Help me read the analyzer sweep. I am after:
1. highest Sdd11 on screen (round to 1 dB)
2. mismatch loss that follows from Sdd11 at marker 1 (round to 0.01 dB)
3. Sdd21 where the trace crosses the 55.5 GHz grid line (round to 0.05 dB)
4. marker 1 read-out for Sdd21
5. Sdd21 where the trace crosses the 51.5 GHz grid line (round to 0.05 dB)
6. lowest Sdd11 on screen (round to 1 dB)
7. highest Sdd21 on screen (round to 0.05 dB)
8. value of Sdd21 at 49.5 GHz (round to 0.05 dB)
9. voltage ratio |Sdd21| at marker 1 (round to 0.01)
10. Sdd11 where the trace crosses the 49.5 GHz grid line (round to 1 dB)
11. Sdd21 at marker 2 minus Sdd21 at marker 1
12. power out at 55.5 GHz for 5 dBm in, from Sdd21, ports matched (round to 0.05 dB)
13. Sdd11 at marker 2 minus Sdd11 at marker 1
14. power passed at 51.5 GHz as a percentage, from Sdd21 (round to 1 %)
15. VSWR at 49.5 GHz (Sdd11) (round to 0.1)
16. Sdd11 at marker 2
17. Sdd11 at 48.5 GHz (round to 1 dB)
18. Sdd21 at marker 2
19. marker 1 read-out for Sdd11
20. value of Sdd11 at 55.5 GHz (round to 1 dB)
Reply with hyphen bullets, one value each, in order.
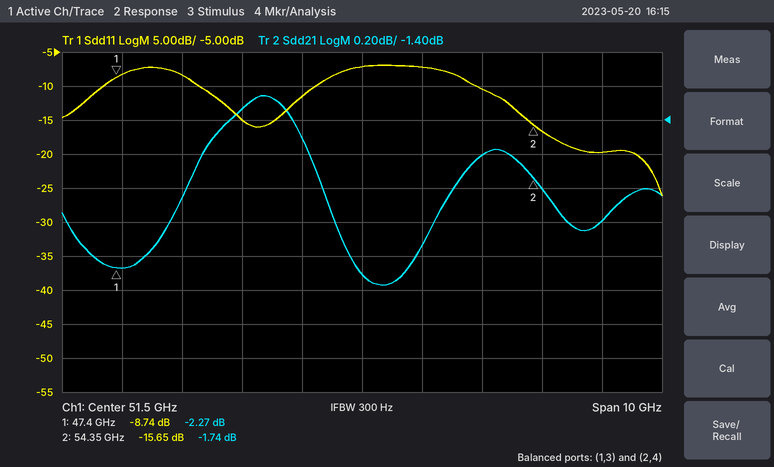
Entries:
- -7 dB
- 0.62 dB
- -2.00 dB
- -2.27 dB
- -2.30 dB
- -26 dB
- -1.25 dB
- -1.35 dB
- 0.77
- -15 dB
- 0.53 dB
- 3.00 dBm
- -6.91 dB
- 59 %
- 1.4
- -15.65 dB
- -8 dB
- -1.74 dB
- -8.74 dB
- -20 dB
